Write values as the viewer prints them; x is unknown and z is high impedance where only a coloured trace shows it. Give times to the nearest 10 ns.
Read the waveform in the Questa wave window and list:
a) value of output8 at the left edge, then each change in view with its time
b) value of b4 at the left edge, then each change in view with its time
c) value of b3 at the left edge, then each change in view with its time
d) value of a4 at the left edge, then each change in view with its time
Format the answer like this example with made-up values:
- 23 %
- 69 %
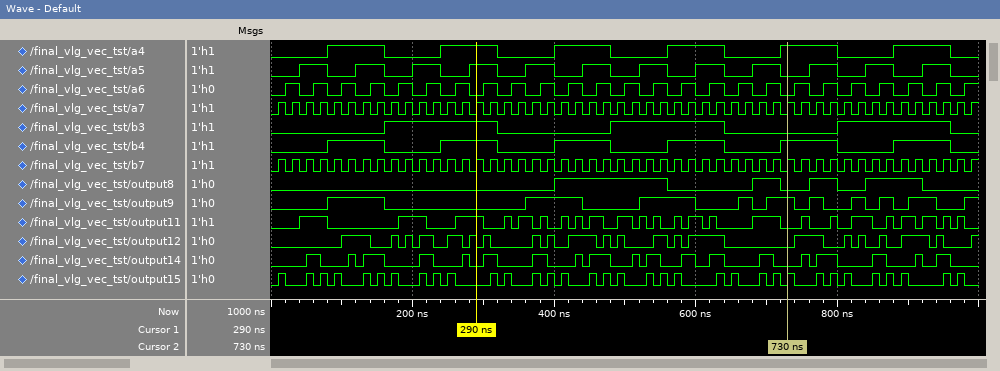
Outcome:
- 0, 1 at 400 ns, 0 at 560 ns, 1 at 680 ns, 0 at 720 ns, 1 at 760 ns, 0 at 800 ns, 1 at 840 ns, 0 at 920 ns
- 0, 1 at 80 ns, 0 at 160 ns, 1 at 240 ns, 0 at 320 ns, 1 at 400 ns, 0 at 480 ns, 1 at 560 ns, 0 at 640 ns, 1 at 720 ns, 0 at 800 ns, 1 at 880 ns, 0 at 960 ns
- 0, 1 at 160 ns, 0 at 320 ns, 1 at 480 ns, 0 at 640 ns, 1 at 800 ns, 0 at 960 ns
- 0, 1 at 80 ns, 0 at 160 ns, 1 at 240 ns, 0 at 320 ns, 1 at 400 ns, 0 at 480 ns, 1 at 560 ns, 0 at 640 ns, 1 at 720 ns, 0 at 800 ns, 1 at 880 ns, 0 at 960 ns
